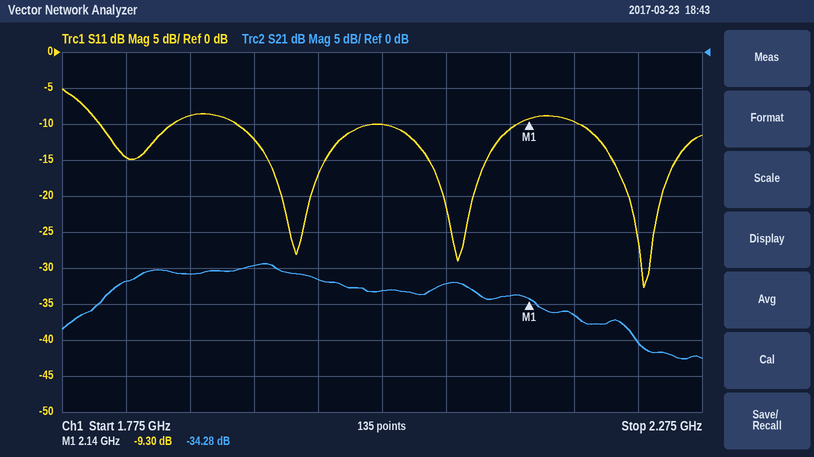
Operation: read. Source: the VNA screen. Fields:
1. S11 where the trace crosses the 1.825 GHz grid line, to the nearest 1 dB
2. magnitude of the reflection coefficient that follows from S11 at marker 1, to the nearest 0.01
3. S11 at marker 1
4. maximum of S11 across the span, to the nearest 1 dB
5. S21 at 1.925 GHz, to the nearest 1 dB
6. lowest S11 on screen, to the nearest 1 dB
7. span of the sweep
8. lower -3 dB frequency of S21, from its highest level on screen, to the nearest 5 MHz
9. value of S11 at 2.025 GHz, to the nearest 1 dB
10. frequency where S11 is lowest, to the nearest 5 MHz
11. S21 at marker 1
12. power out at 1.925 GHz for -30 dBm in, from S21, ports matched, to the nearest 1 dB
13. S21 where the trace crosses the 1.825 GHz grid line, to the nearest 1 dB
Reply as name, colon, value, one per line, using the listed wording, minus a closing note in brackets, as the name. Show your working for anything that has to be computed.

S11 where the trace crosses the 1.825 GHz grid line, to the nearest 1 dB: -15 dB
magnitude of the reflection coefficient that follows from S11 at marker 1, to the nearest 0.01: 10^(-9.3/20) ≈ 0.34
S11 at marker 1: -9.30 dB
maximum of S11 across the span, to the nearest 1 dB: -5 dB
S21 at 1.925 GHz, to the nearest 1 dB: -30 dB
lowest S11 on screen, to the nearest 1 dB: -33 dB
span of the sweep: 500 MHz
lower -3 dB frequency of S21, from its highest level on screen, to the nearest 5 MHz: 1.820 GHz
value of S11 at 2.025 GHz, to the nearest 1 dB: -10 dB
frequency where S11 is lowest, to the nearest 5 MHz: 2.230 GHz
S21 at marker 1: -34.28 dB
power out at 1.925 GHz for -30 dBm in, from S21, ports matched, to the nearest 1 dB: -30 dBm + (-30 dB) = -60 dBm
S21 where the trace crosses the 1.825 GHz grid line, to the nearest 1 dB: -32 dB
